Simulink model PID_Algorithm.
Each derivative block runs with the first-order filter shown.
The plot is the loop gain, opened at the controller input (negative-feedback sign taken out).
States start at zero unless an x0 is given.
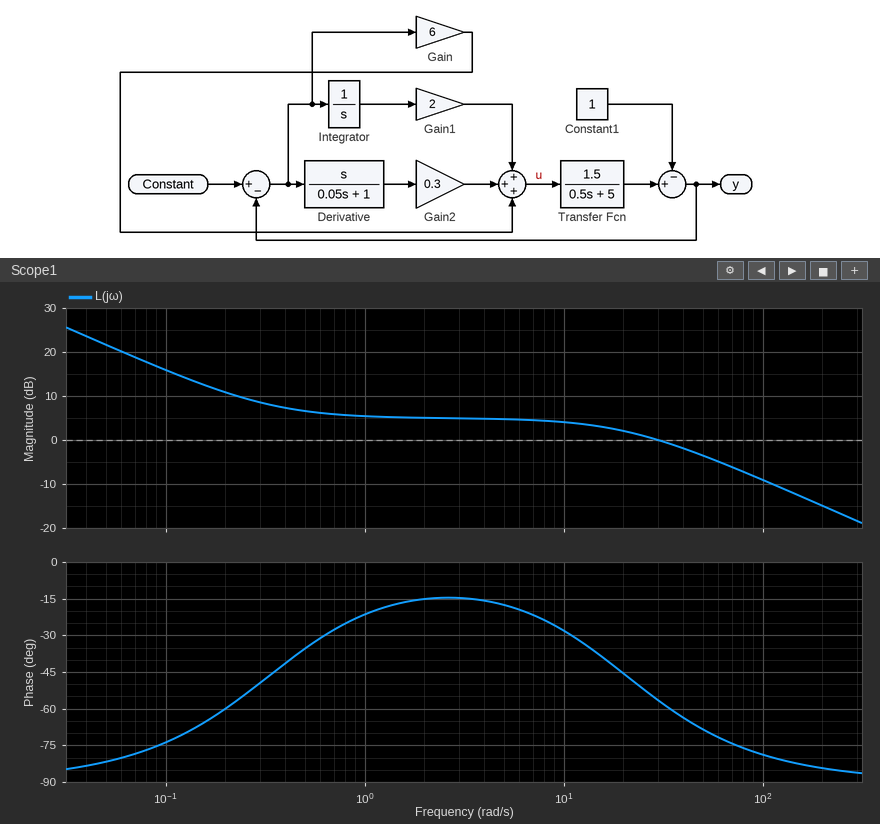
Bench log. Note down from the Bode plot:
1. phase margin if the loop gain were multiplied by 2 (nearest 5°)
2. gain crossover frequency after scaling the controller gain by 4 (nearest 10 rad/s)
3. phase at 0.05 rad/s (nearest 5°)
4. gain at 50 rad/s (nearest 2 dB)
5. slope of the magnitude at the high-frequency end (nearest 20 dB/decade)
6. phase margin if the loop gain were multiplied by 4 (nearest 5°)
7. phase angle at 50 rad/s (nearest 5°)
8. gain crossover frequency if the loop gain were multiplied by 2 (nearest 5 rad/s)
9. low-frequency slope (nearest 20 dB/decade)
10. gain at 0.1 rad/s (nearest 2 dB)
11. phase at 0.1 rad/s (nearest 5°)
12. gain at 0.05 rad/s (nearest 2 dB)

105°
140 rad/s
-80°
-4 dB
-20 dB/decade
100°
-70°
70 rad/s
-20 dB/decade
16 dB
-75°
22 dB
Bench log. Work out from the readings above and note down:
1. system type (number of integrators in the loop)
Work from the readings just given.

1
